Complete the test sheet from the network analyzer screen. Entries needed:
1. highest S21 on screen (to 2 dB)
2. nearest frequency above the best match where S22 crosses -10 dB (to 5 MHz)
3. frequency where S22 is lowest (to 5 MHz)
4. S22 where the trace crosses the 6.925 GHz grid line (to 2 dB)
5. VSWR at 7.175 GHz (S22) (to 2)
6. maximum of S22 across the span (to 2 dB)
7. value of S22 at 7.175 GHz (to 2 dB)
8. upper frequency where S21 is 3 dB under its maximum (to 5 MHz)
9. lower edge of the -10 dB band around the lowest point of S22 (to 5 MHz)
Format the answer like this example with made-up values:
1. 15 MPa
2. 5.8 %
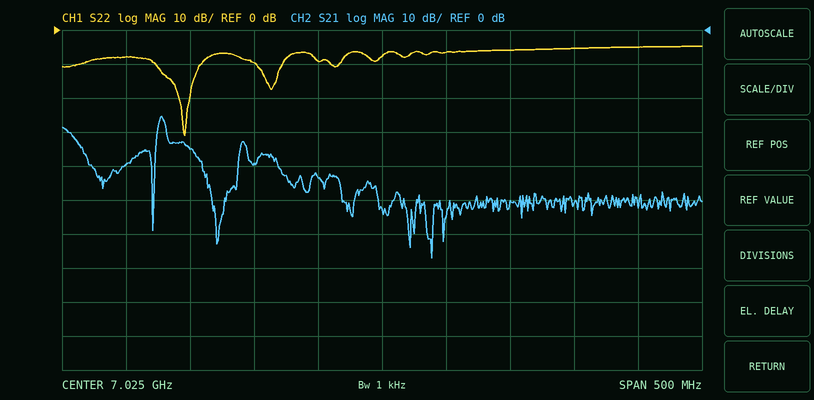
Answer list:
1. -26 dB
2. 6.885 GHz
3. 6.870 GHz
4. -10 dB
5. 4
6. -4 dB
7. -6 dB
8. 6.855 GHz
9. 6.850 GHz
